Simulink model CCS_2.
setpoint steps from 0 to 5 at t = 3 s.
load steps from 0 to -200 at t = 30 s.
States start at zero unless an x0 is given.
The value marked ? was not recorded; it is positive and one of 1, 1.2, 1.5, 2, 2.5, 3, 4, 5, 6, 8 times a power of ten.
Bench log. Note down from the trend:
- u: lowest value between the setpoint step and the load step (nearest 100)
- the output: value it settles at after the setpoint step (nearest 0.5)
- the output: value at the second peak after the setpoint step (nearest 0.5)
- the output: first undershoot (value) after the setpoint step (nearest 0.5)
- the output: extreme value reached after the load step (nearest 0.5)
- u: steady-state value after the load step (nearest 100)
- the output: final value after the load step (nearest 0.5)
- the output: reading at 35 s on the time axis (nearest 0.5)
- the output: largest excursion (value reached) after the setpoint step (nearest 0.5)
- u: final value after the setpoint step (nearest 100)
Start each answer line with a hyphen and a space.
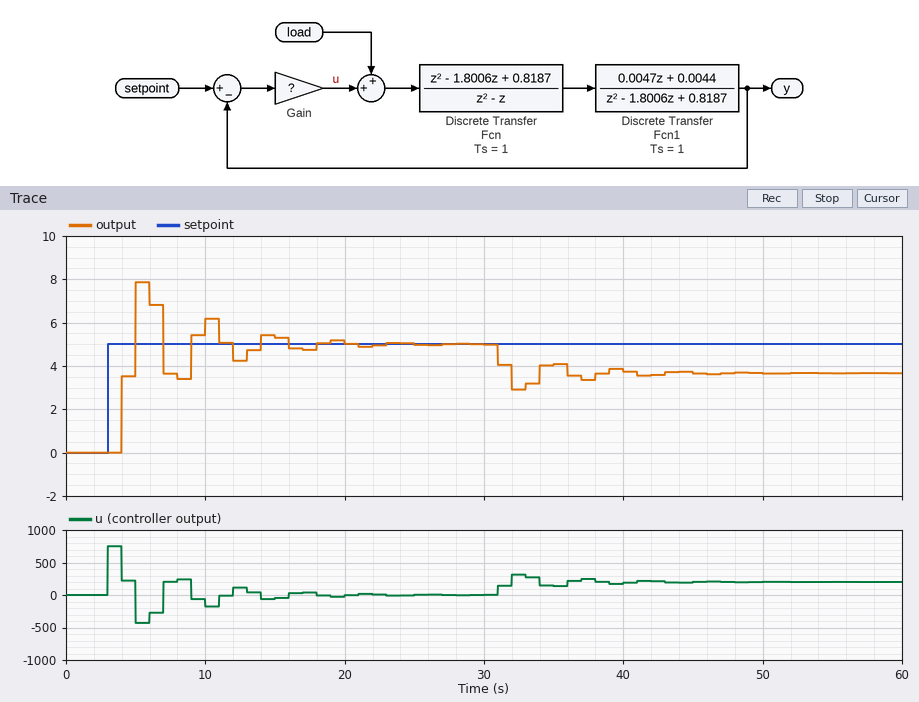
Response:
- -400
- 5.0
- 6.0
- 3.5
- 3.0
- 200
- 3.5
- 4.0
- 8.0
- 0
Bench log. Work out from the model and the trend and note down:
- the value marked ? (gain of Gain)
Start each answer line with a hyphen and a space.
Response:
- 150
